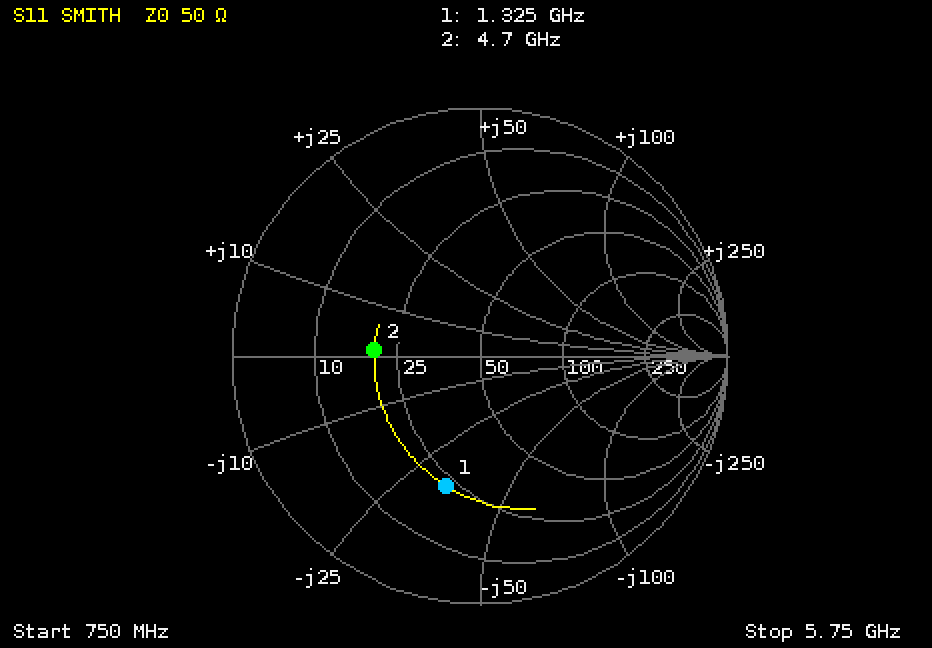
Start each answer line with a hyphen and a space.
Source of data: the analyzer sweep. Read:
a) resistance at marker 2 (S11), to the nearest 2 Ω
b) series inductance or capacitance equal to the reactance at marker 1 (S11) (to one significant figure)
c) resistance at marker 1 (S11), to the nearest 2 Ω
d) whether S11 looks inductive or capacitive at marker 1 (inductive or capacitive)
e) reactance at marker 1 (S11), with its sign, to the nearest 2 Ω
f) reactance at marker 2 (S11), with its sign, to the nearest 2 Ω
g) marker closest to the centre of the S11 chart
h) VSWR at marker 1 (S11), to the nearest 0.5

- 20 Ω
- 4 pF
- 22 Ω
- capacitive
- -34 Ω
- +2 Ω
- marker 2
- 3.5
